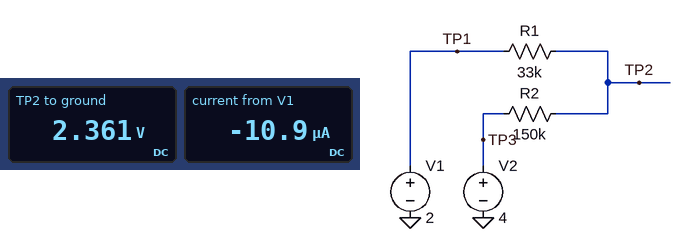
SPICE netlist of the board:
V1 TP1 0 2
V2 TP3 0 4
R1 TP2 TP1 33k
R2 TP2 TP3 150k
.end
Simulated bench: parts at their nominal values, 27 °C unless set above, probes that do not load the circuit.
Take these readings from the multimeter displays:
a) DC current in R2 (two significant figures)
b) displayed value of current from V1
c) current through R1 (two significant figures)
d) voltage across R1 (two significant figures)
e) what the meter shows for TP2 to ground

11 µA
-10.9 µA
11 µA
360 mV
2.361 V
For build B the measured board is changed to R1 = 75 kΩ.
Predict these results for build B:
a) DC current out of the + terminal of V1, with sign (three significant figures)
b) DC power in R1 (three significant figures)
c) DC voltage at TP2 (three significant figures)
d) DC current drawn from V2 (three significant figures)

-8.89 µA
5.93 µW
2.67 V
8.89 µA
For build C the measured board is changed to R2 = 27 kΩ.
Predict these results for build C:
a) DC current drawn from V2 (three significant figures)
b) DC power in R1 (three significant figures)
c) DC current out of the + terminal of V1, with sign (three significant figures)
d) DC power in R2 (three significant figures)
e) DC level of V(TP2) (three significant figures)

33.3 µA
36.7 µW
-33.3 µA
30.0 µW
3.10 V
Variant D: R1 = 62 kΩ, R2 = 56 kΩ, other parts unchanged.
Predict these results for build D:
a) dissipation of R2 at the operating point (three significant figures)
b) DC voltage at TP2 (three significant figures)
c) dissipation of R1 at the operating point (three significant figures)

16.1 µW
3.05 V
17.8 µW
